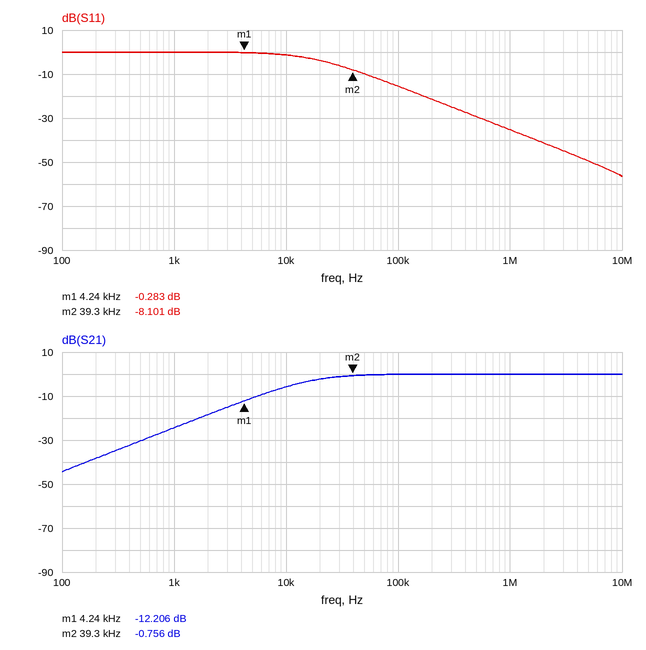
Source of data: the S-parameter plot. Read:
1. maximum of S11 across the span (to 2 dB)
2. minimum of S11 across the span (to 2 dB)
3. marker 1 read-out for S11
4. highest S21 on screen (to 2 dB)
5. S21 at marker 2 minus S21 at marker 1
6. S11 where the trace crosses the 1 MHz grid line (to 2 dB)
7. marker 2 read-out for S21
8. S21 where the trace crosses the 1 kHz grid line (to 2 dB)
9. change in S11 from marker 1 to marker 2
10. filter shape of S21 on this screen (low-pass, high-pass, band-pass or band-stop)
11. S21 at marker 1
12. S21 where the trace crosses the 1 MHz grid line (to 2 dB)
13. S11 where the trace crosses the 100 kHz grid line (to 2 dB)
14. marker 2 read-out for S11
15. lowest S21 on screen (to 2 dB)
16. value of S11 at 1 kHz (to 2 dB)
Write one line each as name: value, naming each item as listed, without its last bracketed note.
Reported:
maximum of S11 across the span: 0 dB
minimum of S11 across the span: -56 dB
marker 1 read-out for S11: -0.283 dB
highest S21 on screen: 0 dB
S21 at marker 2 minus S21 at marker 1: 11.450 dB
S11 where the trace crosses the 1 MHz grid line: -36 dB
marker 2 read-out for S21: -0.756 dB
S21 where the trace crosses the 1 kHz grid line: -24 dB
change in S11 from marker 1 to marker 2: -7.818 dB
filter shape of S21 on this screen: high-pass
S21 at marker 1: -12.206 dB
S21 where the trace crosses the 1 MHz grid line: 0 dB
S11 where the trace crosses the 100 kHz grid line: -16 dB
marker 2 read-out for S11: -8.101 dB
lowest S21 on screen: -44 dB
value of S11 at 1 kHz: 0 dB
